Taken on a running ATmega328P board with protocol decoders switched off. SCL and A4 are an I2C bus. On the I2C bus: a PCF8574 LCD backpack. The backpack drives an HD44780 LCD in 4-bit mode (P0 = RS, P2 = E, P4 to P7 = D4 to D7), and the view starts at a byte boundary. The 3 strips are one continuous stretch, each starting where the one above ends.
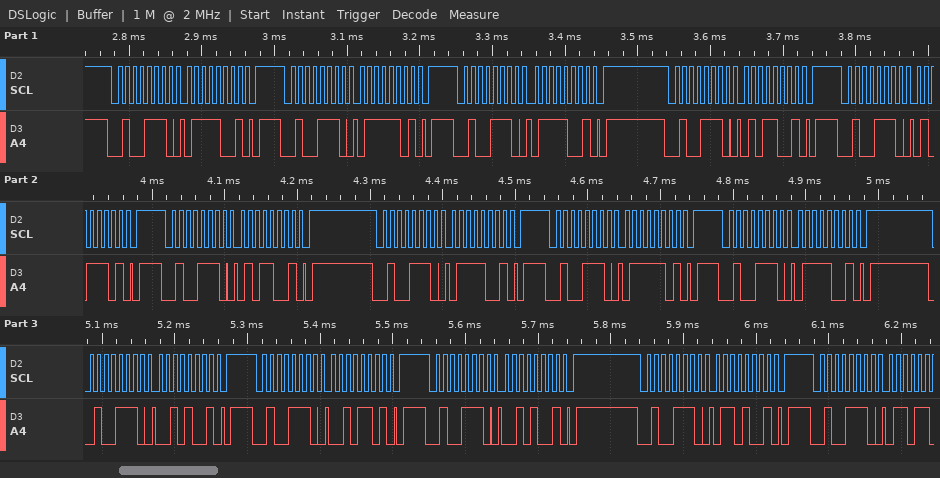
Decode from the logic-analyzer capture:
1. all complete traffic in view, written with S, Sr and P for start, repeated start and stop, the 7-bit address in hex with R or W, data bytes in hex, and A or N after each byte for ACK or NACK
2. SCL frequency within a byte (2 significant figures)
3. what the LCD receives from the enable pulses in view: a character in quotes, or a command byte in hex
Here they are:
S 27W A 79 A P S 27W A 7D A P S 27W A 79 A P S 27W A 59 A P S 27W A 5D A P S 27W A 59 A P S 27W A 79 A P S 27W A 7D A P S 27W A 79 A P S 27W A 29 A P S 27W A 2D A P S 27W A 29 A P S 27W A 69 A P S 27W A
100 kHz
'u' 'r'
